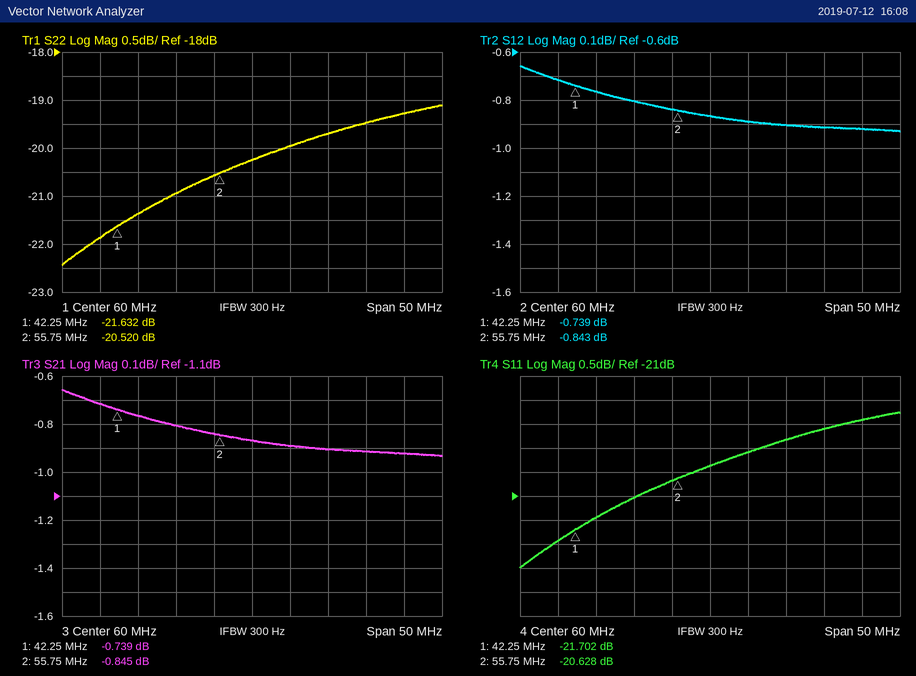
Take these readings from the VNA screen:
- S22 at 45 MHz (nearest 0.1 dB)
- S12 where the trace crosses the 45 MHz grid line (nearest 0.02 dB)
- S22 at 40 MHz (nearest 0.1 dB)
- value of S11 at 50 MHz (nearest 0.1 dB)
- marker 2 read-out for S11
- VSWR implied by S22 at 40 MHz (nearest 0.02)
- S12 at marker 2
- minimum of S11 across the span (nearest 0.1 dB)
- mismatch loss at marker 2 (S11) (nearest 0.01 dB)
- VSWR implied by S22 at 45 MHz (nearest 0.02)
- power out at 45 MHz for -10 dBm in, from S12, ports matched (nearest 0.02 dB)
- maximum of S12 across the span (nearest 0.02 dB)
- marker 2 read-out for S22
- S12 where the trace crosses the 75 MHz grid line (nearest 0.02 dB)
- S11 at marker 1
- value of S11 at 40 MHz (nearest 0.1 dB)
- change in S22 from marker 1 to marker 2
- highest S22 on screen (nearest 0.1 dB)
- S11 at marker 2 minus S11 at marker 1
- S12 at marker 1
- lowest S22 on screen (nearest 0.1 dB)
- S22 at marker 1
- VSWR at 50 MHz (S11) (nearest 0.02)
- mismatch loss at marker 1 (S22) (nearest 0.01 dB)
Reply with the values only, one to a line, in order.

-21.4 dB
-0.76 dB
-21.9 dB
-21.0 dB
-20.628 dB
1.18
-0.843 dB
-22.5 dB
0.04 dB
1.18
-10.76 dBm
-0.66 dB
-20.520 dB
-0.92 dB
-21.702 dB
-21.9 dB
1.112 dB
-19.1 dB
1.074 dB
-0.739 dB
-22.4 dB
-21.632 dB
1.20
0.03 dB
